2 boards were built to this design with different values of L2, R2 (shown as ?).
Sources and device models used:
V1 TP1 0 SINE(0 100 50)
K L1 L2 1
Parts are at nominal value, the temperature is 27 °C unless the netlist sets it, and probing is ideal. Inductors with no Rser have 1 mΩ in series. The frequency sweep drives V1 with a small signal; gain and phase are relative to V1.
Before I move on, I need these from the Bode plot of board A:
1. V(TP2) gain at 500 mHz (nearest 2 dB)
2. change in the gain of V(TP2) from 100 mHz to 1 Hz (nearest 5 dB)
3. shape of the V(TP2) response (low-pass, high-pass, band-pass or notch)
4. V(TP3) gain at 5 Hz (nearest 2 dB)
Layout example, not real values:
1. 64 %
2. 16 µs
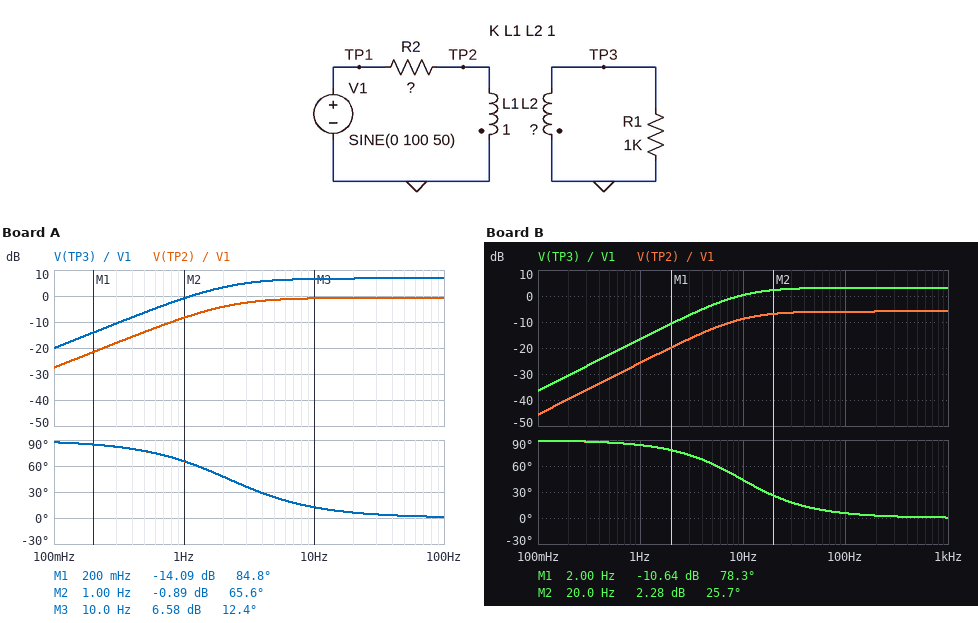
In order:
1. -14 dB
2. 20 dB
3. high-pass
4. 6 dB
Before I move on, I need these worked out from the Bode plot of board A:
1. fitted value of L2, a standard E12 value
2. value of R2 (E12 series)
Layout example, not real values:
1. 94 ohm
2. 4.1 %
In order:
1. 5.6 H
2. 15 Ω
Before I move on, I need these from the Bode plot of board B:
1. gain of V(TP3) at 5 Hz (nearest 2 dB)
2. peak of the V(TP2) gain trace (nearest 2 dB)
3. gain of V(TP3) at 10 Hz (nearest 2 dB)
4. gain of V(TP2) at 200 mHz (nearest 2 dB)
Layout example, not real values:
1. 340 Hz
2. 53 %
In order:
1. -4 dB
2. -6 dB
3. 0 dB
4. -40 dB
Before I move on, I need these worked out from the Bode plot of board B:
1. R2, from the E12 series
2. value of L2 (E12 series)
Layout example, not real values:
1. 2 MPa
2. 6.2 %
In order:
1. 120 Ω
2. 8.2 H
